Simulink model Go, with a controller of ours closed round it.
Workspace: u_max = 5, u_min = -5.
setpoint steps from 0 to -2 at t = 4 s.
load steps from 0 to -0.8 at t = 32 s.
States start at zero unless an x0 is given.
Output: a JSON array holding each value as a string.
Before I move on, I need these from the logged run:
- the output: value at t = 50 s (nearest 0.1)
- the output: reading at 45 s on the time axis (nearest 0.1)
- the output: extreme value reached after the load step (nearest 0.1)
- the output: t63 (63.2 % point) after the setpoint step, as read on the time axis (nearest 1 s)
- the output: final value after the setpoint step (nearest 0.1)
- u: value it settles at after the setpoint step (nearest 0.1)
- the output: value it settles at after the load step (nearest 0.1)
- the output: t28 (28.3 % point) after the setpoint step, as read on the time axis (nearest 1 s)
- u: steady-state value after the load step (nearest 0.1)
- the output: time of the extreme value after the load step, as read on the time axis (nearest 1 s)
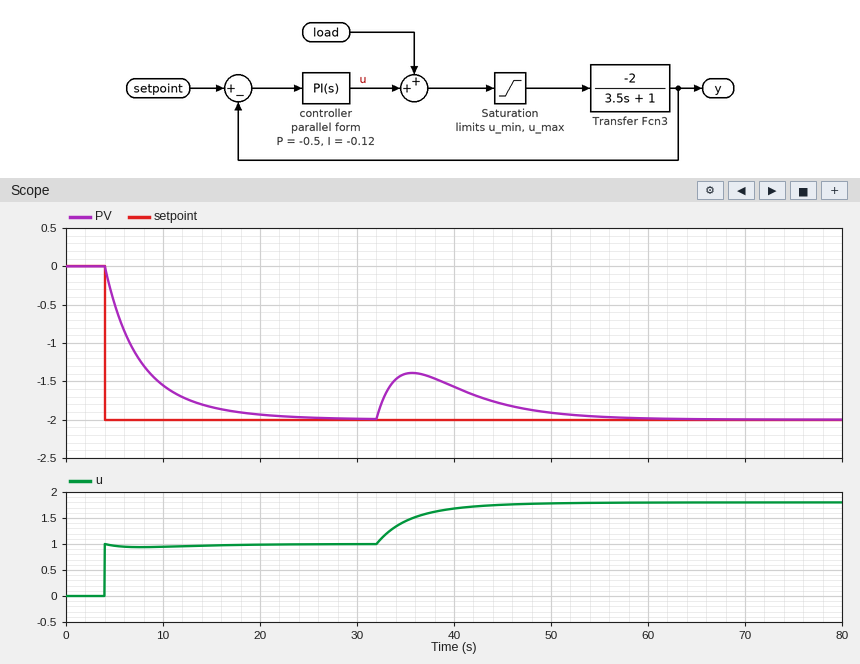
["-1.9", "-1.8", "-1.4", "8 s", "-2.0", "1.0", "-2.0", "5 s", "1.8", "36 s"]
